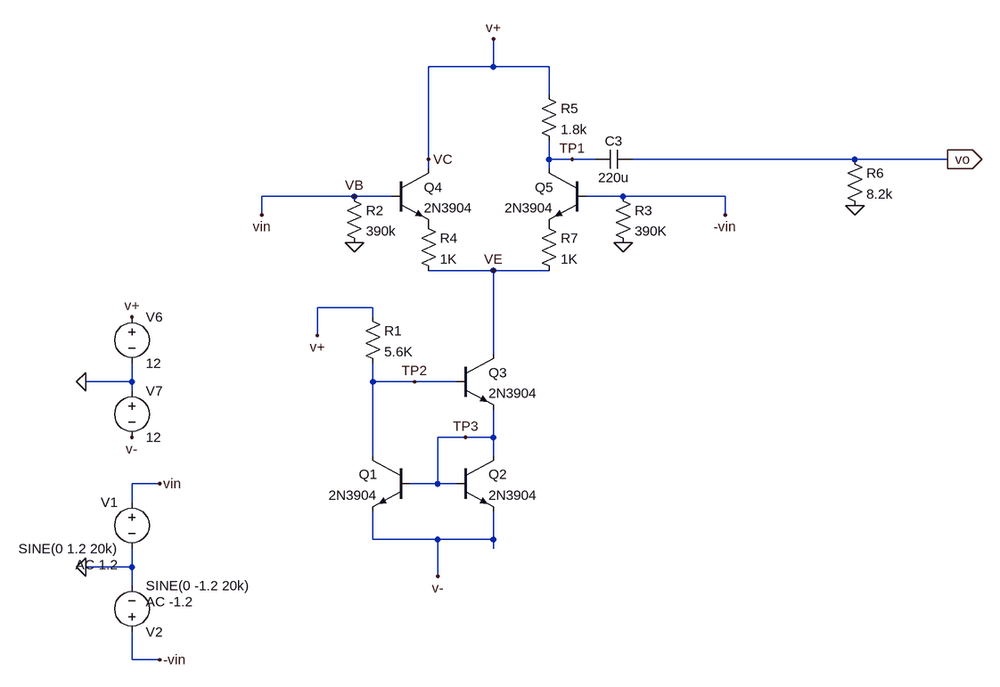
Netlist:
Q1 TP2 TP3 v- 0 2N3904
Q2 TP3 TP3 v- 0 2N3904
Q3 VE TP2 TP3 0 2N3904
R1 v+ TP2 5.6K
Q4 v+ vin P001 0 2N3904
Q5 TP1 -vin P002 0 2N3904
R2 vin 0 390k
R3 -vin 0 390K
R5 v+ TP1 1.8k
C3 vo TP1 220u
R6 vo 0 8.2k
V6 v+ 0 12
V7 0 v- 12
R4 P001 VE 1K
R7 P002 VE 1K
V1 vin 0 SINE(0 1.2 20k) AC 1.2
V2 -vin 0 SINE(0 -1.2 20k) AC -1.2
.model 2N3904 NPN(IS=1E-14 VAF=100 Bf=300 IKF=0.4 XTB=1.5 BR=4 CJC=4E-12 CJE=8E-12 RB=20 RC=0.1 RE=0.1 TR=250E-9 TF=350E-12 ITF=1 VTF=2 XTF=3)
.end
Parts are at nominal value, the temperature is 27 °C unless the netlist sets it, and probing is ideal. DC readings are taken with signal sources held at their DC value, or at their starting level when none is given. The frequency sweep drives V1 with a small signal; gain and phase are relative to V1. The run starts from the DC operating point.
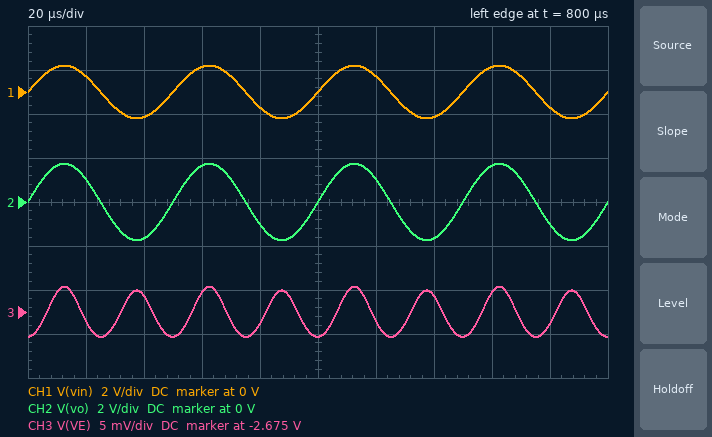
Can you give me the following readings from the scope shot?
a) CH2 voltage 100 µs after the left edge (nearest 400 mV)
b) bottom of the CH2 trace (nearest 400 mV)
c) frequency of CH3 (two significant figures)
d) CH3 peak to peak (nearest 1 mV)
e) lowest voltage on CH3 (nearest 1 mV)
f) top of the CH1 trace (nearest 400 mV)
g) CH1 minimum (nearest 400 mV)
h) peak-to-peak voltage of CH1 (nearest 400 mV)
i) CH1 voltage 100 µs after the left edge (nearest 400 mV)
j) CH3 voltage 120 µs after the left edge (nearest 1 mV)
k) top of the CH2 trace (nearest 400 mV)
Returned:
0 V
-1.6 V
40 kHz
6 mV
-2.678 V
1.2 V
-1.2 V
2.4 V
0 V
-2.676 V
1.6 V
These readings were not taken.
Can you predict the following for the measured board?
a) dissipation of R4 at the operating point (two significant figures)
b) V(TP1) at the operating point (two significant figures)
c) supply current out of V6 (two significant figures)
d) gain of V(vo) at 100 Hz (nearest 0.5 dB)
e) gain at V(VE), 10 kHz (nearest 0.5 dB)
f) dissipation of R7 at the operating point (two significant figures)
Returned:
4.0 mW
8.4 V
8.0 mA
4.0 dB
-20.0 dB
4.0 mW
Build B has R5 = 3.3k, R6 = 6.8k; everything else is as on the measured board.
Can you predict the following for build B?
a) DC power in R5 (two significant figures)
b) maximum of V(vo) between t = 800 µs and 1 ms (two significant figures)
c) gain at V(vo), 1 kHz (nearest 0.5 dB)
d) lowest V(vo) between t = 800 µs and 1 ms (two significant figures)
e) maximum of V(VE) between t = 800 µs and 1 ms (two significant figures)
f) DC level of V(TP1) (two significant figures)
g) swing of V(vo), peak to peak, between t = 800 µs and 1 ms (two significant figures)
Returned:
13 mW
2.6 V
7.5 dB
-2.6 V
-2.7 V
5.4 V
5.2 V
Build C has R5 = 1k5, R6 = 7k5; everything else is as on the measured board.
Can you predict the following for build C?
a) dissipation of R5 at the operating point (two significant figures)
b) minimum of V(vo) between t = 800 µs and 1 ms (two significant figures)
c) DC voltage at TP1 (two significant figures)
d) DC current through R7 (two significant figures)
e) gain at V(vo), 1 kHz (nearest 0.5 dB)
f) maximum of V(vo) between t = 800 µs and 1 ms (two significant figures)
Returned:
6.0 mW
-1.5 V
9.0 V
2.0 mA
2.5 dB
1.5 V
